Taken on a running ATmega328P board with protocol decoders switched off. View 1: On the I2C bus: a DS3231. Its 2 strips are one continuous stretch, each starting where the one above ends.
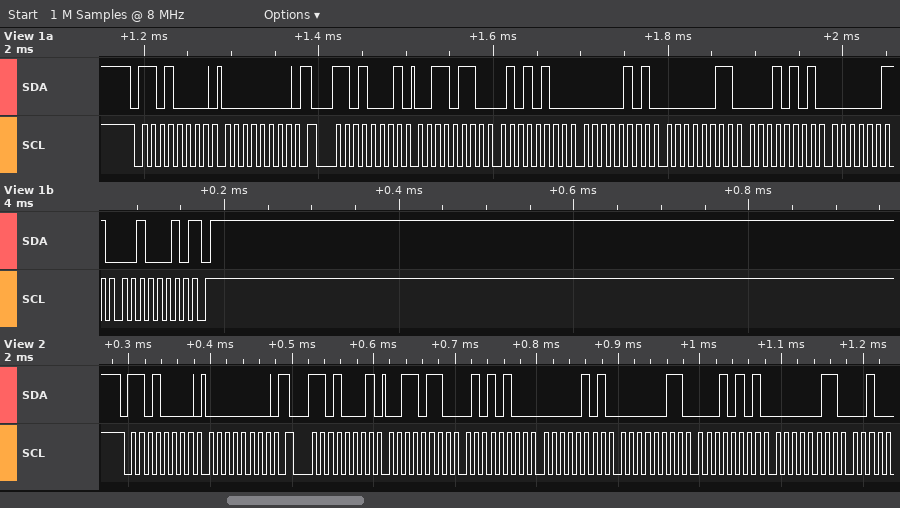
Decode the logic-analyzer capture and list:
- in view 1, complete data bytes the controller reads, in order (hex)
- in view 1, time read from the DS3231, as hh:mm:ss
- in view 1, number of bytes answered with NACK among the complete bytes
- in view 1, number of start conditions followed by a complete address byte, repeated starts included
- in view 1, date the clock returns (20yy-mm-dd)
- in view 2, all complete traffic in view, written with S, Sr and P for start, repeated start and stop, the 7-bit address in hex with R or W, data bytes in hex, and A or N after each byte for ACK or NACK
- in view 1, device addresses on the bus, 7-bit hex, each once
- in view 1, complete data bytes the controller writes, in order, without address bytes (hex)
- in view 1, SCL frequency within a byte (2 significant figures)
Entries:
36 54 05 03 15 03 22
05:54:36
1
2
2022-03-15
S 68W A 00 A Sr 68R A 36 A 54 A 05 A 03 A 15 A 03 A
0x68
00
100 kHz
